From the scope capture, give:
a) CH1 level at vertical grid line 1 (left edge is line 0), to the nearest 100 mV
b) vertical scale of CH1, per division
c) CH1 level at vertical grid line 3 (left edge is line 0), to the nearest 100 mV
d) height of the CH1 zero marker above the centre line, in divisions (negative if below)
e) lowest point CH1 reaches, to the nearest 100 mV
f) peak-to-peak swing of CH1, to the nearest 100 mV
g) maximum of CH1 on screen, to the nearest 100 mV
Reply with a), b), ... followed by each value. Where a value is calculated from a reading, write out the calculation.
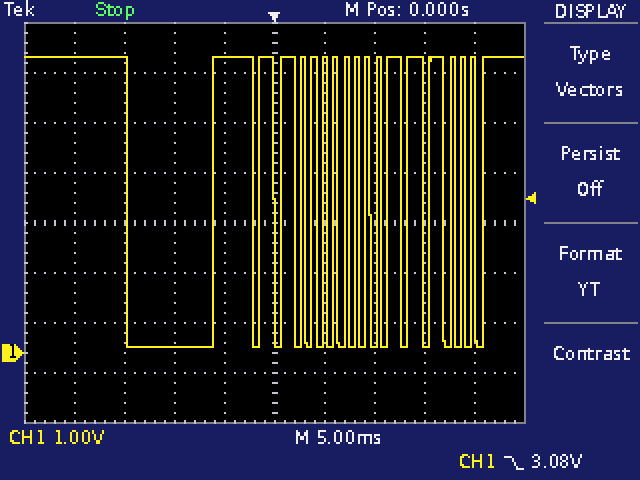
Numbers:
a) 5.9 V
b) 1 V
c) 100 mV
d) -2.6 div
e) 100 mV
f) 5.9 V − (100 mV) = 5.8 V
g) 5.9 V
